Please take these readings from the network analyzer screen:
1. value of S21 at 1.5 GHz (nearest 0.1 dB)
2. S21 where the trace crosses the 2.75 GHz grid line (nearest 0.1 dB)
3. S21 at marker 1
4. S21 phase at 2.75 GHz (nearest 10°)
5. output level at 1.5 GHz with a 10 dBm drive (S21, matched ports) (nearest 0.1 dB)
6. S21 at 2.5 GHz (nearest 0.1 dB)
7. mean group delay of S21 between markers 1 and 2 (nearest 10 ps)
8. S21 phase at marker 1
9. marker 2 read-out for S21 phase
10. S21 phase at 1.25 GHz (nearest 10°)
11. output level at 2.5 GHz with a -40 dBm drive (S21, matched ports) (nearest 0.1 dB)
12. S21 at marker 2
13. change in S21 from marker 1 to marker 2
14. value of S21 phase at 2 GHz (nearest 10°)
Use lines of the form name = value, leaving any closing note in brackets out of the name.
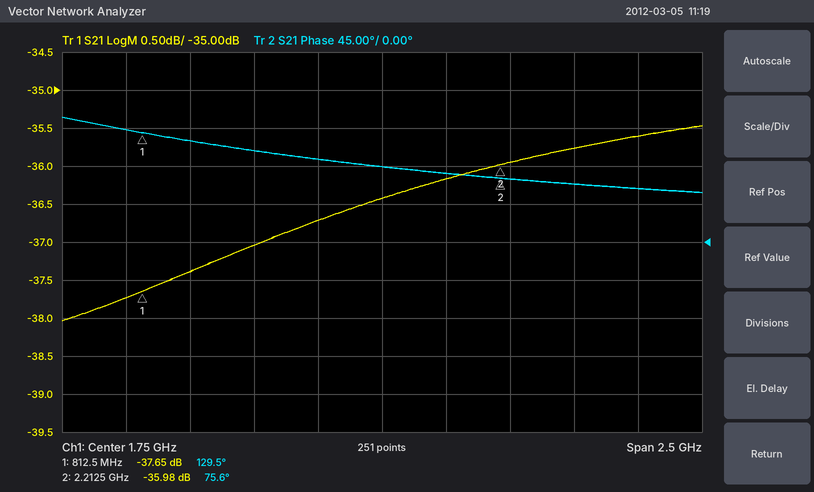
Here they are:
value of S21 at 1.5 GHz = -36.7 dB
S21 where the trace crosses the 2.75 GHz grid line = -35.6 dB
S21 at marker 1 = -37.65 dB
S21 phase at 2.75 GHz = 60°
output level at 1.5 GHz with a 10 dBm drive (S21, matched ports) = -26.7 dBm
S21 at 2.5 GHz = -35.8 dB
mean group delay of S21 between markers 1 and 2 = 110 ps
S21 phase at marker 1 = 129.5°
marker 2 read-out for S21 phase = 75.6°
S21 phase at 1.25 GHz = 110°
output level at 2.5 GHz with a -40 dBm drive (S21, matched ports) = -75.8 dBm
S21 at marker 2 = -35.98 dB
change in S21 from marker 1 to marker 2 = 1.67 dB
value of S21 phase at 2 GHz = 80°
